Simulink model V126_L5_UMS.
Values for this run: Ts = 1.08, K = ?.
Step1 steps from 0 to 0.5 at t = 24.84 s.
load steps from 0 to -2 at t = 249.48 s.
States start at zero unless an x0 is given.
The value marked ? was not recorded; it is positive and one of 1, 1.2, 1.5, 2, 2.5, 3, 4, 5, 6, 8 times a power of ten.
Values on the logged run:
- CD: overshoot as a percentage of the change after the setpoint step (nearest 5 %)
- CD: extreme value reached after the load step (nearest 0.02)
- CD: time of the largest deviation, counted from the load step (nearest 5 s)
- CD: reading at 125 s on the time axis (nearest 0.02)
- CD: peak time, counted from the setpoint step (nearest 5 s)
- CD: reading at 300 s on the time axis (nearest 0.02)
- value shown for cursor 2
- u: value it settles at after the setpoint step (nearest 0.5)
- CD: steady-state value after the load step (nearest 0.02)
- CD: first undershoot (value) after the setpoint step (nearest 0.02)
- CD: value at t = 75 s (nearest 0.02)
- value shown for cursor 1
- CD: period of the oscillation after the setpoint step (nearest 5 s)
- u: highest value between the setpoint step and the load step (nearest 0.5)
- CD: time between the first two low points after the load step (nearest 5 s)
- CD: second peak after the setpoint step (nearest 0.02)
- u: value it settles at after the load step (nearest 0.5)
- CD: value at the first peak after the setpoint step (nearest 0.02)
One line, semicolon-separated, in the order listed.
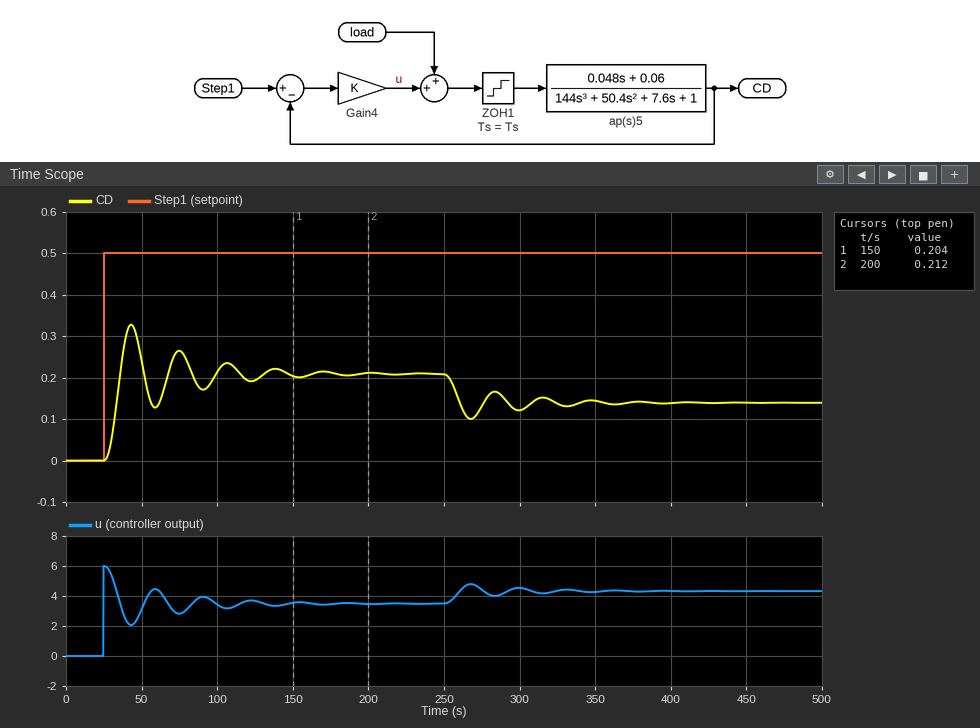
55 %; 0.10; 20 s; 0.20; 20 s; 0.12; 0.212; 3.5; 0.14; 0.12; 0.26; 0.204; 30 s; 6.0; 30 s; 0.26; 4.5; 0.32
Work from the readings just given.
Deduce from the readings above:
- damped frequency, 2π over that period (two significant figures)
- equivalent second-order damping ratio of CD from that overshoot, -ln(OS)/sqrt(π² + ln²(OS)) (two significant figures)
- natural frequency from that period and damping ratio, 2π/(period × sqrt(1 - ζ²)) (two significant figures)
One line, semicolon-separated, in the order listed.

0.21 rad/s; 0.19; 0.21 rad/s
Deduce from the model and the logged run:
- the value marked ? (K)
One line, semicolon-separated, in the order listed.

12
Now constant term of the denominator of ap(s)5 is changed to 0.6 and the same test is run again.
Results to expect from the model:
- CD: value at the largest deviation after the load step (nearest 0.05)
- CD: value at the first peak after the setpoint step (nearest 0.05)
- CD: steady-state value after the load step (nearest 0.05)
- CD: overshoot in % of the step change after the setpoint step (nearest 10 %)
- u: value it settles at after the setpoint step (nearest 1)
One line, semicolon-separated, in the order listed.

0.15; 0.40; 0.20; 40 %; 3
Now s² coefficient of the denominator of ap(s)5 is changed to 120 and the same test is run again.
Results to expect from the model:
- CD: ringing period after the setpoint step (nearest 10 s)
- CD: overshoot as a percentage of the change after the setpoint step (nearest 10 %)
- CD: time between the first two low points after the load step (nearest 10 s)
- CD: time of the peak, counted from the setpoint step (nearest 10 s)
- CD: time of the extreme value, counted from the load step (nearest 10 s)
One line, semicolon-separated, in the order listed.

50 s; 50 %; 50 s; 30 s; 30 s
